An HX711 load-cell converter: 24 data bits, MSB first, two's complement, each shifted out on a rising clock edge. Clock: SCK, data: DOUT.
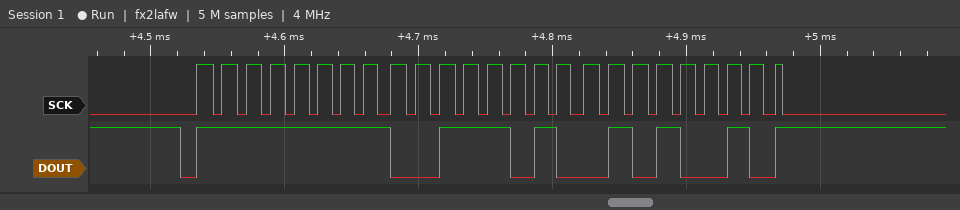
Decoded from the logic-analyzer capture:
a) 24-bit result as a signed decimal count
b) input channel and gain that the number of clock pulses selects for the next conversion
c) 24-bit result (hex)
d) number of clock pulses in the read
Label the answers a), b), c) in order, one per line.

a) -50606
b) channel A, gain 128
c) 0xFF3A52
d) 25
